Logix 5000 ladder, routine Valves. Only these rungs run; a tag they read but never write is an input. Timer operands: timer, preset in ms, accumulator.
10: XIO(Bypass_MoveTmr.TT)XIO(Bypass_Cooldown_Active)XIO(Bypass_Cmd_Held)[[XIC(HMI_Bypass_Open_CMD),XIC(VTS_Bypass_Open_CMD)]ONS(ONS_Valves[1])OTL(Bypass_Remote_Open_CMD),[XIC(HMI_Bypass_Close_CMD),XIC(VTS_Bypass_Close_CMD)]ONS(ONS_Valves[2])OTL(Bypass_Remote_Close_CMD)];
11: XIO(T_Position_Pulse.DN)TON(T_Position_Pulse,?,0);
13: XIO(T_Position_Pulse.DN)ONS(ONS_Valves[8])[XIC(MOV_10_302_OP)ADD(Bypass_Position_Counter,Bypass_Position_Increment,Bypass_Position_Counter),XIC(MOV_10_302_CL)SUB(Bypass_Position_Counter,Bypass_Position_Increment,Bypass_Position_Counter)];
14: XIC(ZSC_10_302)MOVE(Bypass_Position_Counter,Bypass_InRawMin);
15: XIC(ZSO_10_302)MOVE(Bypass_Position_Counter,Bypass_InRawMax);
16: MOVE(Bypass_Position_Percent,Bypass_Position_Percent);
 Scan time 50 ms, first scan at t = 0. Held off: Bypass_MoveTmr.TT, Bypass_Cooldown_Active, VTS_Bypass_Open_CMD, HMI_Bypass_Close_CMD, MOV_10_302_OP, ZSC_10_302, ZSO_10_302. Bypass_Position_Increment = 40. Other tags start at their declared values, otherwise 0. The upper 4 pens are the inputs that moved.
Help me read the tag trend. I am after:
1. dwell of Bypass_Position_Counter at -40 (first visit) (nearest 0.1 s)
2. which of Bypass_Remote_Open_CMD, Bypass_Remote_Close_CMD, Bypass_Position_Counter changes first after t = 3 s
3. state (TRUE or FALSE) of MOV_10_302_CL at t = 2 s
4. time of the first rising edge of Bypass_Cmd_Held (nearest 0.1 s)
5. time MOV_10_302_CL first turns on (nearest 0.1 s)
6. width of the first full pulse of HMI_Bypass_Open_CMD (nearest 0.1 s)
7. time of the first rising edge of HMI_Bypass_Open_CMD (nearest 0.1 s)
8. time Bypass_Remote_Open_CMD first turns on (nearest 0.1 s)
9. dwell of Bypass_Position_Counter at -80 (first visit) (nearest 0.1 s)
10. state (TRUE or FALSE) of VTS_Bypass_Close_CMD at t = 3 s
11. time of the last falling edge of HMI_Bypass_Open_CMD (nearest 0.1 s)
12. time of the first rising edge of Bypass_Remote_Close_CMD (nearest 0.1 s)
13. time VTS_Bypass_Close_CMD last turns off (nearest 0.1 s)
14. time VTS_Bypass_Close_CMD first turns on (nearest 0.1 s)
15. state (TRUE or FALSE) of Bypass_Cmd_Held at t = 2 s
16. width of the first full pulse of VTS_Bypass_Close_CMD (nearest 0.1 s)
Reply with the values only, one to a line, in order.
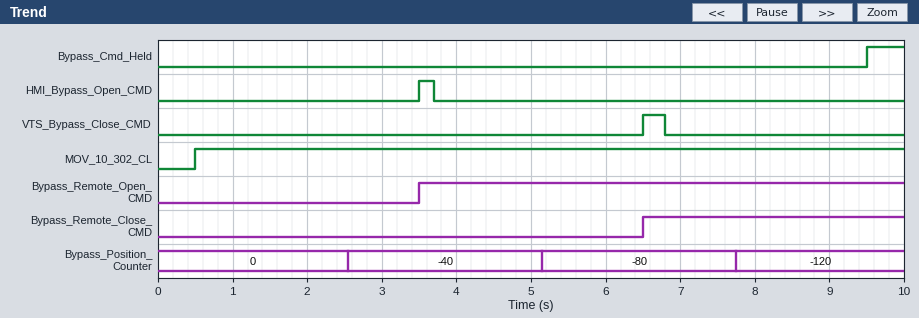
2.6 s
Bypass_Remote_Open_CMD
TRUE
9.5 s
0.5 s
0.2 s
3.5 s
3.5 s
2.6 s
FALSE
3.7 s
6.5 s
6.8 s
6.5 s
FALSE
0.3 s
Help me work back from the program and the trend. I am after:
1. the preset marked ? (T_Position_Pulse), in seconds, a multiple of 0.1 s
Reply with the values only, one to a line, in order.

2.5 s
